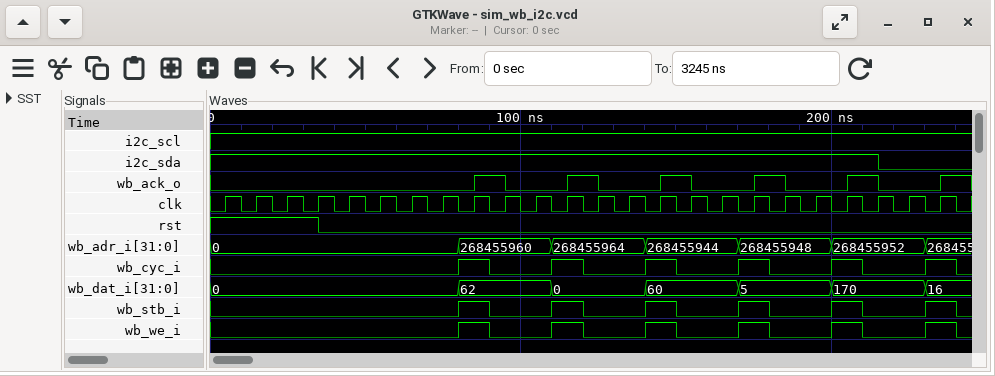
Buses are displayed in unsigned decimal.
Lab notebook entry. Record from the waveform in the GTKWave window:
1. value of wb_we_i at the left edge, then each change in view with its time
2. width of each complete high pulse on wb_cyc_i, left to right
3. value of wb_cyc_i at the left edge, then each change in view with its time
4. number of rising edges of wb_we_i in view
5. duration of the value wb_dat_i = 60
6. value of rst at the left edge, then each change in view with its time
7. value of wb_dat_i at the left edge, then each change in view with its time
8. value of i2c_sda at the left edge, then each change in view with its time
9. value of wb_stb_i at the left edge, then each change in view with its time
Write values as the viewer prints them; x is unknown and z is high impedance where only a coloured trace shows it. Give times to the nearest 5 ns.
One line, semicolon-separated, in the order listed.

0, 1 at 80 ns, 0 at 90 ns, 1 at 110 ns, 0 at 120 ns, 1 at 140 ns, 0 at 150 ns, 1 at 170 ns, 0 at 180 ns, 1 at 200 ns, 0 at 210 ns, 1 at 230 ns, 0 at 240 ns; 10 ns, 10 ns, 10 ns, 10 ns, 10 ns, 10 ns; 0, 1 at 80 ns, 0 at 90 ns, 1 at 110 ns, 0 at 120 ns, 1 at 140 ns, 0 at 150 ns, 1 at 170 ns, 0 at 180 ns, 1 at 200 ns, 0 at 210 ns, 1 at 230 ns, 0 at 240 ns; 6; 30 ns; 1, 0 at 35 ns; 0, 62 at 80 ns, 0 at 110 ns, 60 at 140 ns, 5 at 170 ns, 170 at 200 ns, 16 at 230 ns; 1, 0 at 215 ns; 0, 1 at 80 ns, 0 at 90 ns, 1 at 110 ns, 0 at 120 ns, 1 at 140 ns, 0 at 150 ns, 1 at 170 ns, 0 at 180 ns, 1 at 200 ns, 0 at 210 ns, 1 at 230 ns, 0 at 240 ns
